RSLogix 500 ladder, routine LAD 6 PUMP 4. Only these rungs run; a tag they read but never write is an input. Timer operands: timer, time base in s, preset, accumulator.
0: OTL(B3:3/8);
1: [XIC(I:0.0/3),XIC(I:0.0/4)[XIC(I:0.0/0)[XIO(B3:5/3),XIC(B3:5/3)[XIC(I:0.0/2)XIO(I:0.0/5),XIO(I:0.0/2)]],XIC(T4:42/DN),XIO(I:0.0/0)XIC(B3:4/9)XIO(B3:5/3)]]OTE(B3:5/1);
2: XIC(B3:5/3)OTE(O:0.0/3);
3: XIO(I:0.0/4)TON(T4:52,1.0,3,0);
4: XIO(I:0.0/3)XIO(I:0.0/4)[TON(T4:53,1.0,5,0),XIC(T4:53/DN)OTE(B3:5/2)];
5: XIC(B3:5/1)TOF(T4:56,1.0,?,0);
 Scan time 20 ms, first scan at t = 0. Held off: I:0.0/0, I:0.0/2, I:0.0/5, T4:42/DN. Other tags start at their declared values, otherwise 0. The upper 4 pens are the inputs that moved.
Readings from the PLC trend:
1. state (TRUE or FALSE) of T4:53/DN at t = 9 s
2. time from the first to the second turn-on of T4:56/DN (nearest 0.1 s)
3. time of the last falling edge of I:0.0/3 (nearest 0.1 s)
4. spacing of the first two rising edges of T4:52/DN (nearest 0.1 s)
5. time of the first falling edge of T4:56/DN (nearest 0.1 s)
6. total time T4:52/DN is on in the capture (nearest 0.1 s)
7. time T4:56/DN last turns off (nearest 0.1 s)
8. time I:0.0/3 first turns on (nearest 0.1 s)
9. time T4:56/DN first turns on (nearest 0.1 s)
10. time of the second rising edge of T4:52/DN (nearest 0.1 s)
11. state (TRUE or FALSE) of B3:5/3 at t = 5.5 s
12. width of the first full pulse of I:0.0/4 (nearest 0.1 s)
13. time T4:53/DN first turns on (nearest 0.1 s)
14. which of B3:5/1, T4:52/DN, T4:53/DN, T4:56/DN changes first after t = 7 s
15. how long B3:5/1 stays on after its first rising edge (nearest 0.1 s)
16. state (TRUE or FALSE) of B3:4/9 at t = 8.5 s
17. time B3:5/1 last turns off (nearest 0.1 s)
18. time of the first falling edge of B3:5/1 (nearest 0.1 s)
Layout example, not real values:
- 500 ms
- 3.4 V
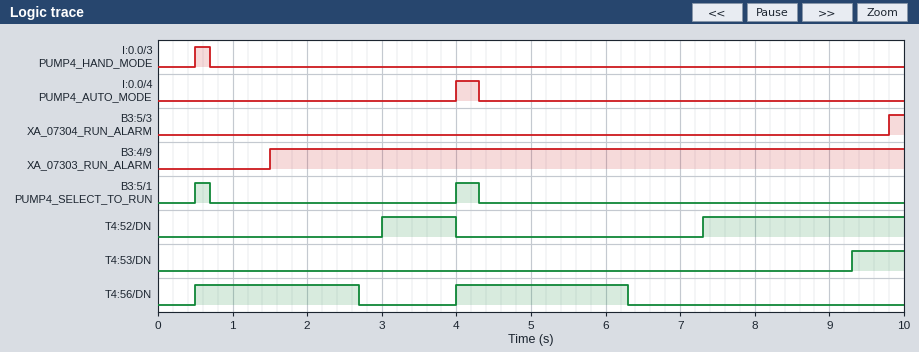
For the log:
- FALSE
- 3.5 s
- 0.7 s
- 4.3 s
- 2.7 s
- 3.7 s
- 6.3 s
- 0.5 s
- 0.5 s
- 7.3 s
- FALSE
- 0.3 s
- 9.3 s
- T4:52/DN
- 0.2 s
- TRUE
- 4.3 s
- 0.7 s
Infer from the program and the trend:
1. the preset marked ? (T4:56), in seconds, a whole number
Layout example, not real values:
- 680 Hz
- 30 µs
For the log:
- 2 s
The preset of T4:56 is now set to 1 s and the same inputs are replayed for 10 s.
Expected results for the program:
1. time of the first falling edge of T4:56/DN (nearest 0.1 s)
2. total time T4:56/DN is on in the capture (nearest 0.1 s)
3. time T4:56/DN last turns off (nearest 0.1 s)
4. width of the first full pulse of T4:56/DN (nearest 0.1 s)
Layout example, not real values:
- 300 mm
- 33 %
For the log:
- 1.7 s
- 2.5 s
- 5.3 s
- 1.2 s
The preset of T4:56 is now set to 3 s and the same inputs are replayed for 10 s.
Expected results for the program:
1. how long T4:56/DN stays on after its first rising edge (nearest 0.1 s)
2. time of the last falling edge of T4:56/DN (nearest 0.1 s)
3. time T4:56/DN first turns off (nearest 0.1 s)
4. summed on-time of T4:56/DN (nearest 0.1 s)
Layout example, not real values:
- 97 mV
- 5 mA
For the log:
- 3.2 s
- 7.3 s
- 3.7 s
- 6.5 s
